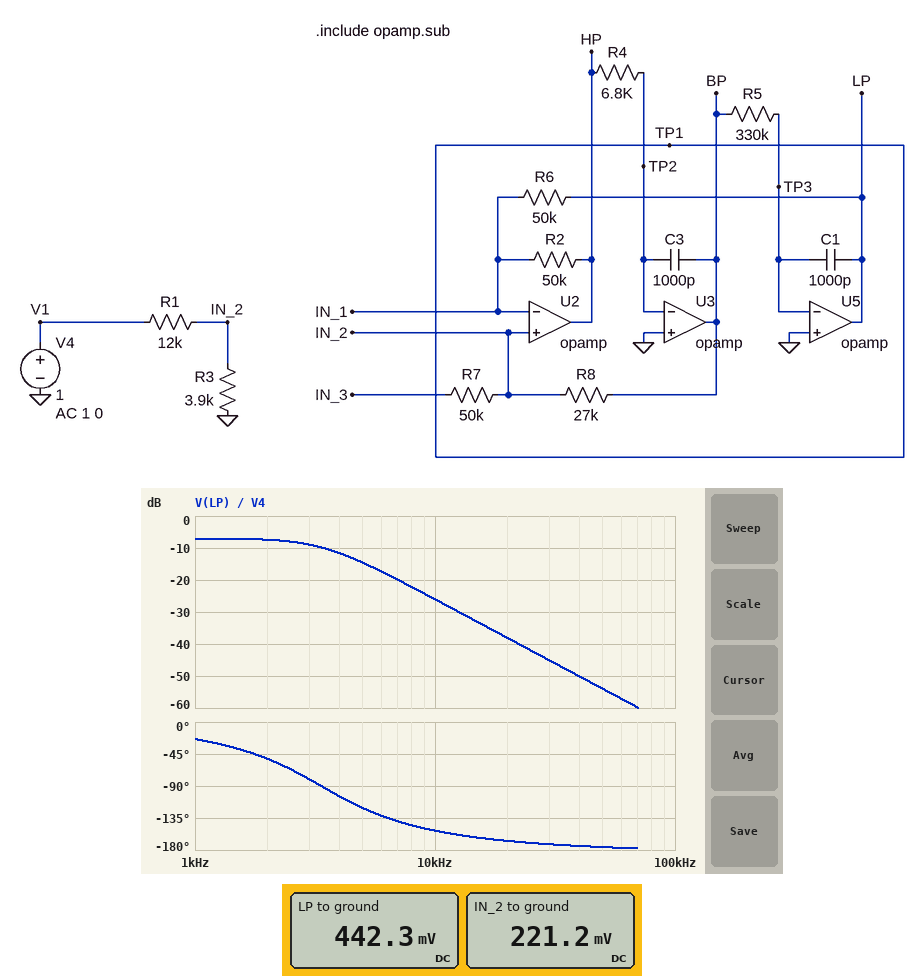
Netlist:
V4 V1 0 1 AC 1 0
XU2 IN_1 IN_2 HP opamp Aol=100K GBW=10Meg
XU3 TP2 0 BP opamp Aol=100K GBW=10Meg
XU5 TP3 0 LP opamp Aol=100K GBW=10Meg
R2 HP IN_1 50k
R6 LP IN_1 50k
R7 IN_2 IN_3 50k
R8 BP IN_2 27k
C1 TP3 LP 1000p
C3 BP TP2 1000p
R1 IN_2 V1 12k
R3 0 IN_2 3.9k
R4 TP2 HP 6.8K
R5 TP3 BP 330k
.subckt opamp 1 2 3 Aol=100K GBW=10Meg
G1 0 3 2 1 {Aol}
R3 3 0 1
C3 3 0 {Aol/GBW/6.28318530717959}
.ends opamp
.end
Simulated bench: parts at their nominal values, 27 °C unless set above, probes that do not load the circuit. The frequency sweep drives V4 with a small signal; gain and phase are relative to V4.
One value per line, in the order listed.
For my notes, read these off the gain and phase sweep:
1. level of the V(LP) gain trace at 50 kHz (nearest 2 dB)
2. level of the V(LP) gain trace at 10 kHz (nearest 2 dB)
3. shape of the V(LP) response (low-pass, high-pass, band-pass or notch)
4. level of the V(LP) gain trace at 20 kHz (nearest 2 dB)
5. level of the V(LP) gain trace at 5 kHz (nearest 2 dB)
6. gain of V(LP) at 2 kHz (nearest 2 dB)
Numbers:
-54 dB
-26 dB
low-pass
-38 dB
-14 dB
-8 dB
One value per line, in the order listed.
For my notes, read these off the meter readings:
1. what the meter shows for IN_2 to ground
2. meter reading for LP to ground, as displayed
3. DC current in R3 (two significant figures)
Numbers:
221.2 mV
442.3 mV
57 µA
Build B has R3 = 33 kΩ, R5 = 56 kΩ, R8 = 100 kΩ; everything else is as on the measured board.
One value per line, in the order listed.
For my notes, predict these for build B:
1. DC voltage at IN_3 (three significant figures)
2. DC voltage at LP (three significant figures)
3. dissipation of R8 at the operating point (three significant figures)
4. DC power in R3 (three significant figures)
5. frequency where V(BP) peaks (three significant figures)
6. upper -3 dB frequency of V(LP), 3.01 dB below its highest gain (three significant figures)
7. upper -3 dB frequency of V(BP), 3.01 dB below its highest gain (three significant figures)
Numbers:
674 mV
1.35 V
4.54 µW
13.8 µW
8.15 kHz
9.44 kHz
10.2 kHz
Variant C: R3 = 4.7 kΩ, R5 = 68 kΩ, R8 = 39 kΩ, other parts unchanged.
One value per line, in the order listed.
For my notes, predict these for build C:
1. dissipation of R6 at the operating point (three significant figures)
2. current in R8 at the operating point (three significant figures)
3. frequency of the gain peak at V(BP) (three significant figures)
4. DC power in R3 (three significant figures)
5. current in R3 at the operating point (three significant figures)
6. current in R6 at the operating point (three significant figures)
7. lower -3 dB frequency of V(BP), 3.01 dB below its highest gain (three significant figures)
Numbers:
1.34 µW
6.64 µA
7.40 kHz
14.3 µW
55.1 µA
5.18 µA
5.77 kHz
